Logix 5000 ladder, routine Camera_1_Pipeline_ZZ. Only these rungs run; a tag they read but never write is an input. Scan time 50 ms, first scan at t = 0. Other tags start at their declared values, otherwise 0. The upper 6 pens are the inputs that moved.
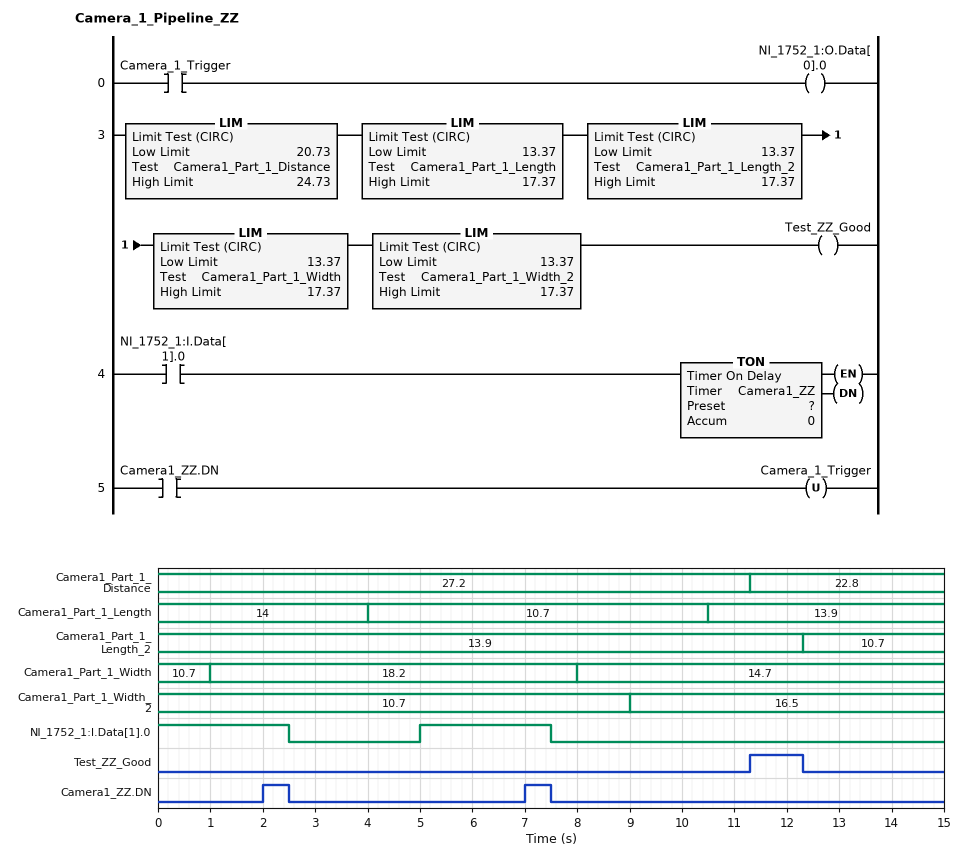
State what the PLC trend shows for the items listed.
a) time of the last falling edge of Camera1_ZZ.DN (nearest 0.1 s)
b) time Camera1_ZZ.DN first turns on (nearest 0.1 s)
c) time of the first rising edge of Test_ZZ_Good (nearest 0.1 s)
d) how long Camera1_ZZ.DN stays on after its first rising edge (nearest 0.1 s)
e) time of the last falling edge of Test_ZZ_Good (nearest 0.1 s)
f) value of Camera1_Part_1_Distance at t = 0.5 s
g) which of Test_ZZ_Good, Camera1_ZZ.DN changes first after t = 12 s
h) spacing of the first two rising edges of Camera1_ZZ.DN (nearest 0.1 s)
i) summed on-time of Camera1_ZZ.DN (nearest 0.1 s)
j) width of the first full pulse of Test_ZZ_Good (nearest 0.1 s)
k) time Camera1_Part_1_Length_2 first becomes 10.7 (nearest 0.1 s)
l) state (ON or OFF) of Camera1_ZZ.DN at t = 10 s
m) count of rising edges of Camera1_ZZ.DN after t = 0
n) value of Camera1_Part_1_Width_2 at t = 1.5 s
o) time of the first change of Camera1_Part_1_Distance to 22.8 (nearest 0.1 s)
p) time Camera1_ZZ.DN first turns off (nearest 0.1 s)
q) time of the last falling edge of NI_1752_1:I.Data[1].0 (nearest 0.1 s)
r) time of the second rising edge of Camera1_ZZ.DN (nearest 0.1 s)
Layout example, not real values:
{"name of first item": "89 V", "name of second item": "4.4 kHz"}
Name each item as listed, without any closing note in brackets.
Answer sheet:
{"time of the last falling edge of Camera1_ZZ.DN": "7.5 s", "time Camera1_ZZ.DN first turns on": "2.0 s", "time of the first rising edge of Test_ZZ_Good": "11.3 s", "how long Camera1_ZZ.DN stays on after its first rising edge": "0.5 s", "time of the last falling edge of Test_ZZ_Good": "12.3 s", "value of Camera1_Part_1_Distance at t = 0.5 s": "27.2", "which of Test_ZZ_Good, Camera1_ZZ.DN changes first after t = 12 s": "Test_ZZ_Good", "spacing of the first two rising edges of Camera1_ZZ.DN": "5.0 s", "summed on-time of Camera1_ZZ.DN": "1.0 s", "width of the first full pulse of Test_ZZ_Good": "1.0 s", "time Camera1_Part_1_Length_2 first becomes 10.7": "12.3 s", "state (ON or OFF) of Camera1_ZZ.DN at t = 10 s": "OFF", "count of rising edges of Camera1_ZZ.DN after t = 0": "2", "value of Camera1_Part_1_Width_2 at t = 1.5 s": "10.7", "time of the first change of Camera1_Part_1_Distance to 22.8": "11.3 s", "time Camera1_ZZ.DN first turns off": "2.5 s", "time of the last falling edge of NI_1752_1:I.Data[1].0": "7.5 s", "time of the second rising edge of Camera1_ZZ.DN": "7.0 s"}
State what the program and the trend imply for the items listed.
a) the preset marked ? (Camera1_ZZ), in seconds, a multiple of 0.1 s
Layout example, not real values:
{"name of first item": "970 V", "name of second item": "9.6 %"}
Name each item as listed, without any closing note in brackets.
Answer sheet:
{"the preset marked ? (Camera1_ZZ), in seconds, a multiple of 0.1 s": "2.0 s"}
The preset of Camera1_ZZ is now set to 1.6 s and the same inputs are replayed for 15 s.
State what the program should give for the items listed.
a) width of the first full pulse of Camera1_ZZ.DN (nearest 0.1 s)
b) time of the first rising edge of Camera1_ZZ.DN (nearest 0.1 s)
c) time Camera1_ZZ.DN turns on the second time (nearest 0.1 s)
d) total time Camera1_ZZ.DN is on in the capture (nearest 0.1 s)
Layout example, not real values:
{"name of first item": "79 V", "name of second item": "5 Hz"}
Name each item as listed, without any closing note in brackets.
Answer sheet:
{"width of the first full pulse of Camera1_ZZ.DN": "0.9 s", "time of the first rising edge of Camera1_ZZ.DN": "1.6 s", "time Camera1_ZZ.DN turns on the second time": "6.6 s", "total time Camera1_ZZ.DN is on in the capture": "1.8 s"}
